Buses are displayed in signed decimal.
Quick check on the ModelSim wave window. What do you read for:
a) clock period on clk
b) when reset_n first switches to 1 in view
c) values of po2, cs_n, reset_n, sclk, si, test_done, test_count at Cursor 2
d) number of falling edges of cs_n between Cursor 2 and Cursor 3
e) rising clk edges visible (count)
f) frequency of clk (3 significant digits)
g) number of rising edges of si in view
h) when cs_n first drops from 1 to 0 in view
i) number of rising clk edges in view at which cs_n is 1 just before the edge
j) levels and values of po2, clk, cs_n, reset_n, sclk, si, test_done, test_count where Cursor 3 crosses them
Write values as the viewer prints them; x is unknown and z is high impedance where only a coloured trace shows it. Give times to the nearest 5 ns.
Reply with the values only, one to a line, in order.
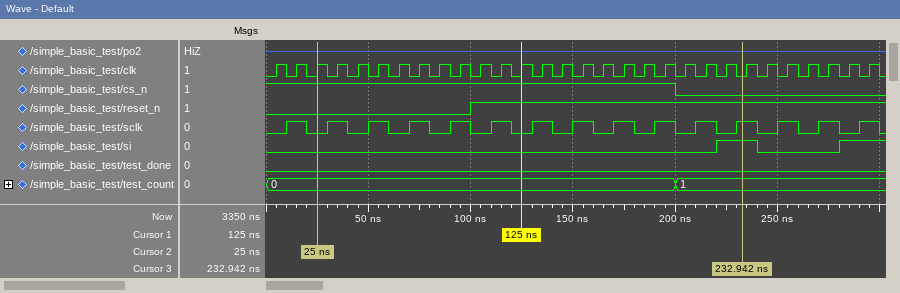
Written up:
10 ns
100 ns
po2=z, cs_n=1, reset_n=0, sclk=0, si=0, test_done=0, test_count=0
1
30
100 MHz
2
200 ns
20
po2=z, clk=0, cs_n=0, reset_n=1, sclk=1, si=1, test_done=0, test_count=1
